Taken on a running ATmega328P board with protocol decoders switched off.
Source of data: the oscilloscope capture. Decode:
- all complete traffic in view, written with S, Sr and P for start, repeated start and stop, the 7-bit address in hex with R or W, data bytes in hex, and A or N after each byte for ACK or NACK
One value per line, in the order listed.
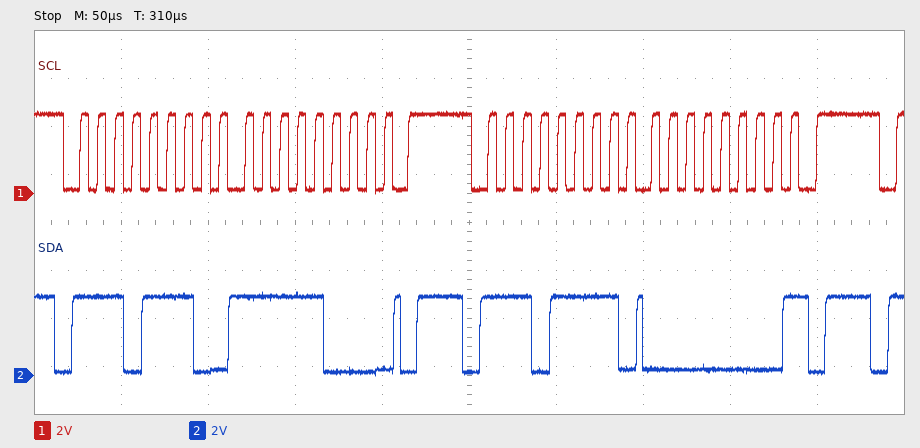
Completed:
S 77W A F8 A P S 77R A 00 N P
